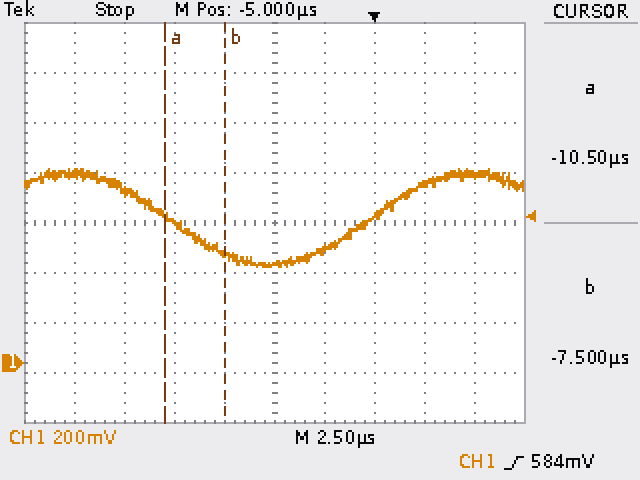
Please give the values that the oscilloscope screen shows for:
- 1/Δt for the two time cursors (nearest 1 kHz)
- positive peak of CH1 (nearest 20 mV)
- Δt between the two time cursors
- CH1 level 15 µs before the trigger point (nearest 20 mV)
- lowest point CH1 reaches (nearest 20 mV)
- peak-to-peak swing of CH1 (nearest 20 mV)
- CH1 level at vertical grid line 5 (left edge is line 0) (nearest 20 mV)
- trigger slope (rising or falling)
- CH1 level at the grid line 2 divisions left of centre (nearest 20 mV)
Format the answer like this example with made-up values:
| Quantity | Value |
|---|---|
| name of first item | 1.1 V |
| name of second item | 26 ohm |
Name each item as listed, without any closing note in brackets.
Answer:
| Quantity | Value |
|---|---|
| 1/Δt for the two time cursors | 333 kHz |
| positive peak of CH1 | 780 mV |
| Δt between the two time cursors | 3.00 µs |
| CH1 level 15 µs before the trigger point | 760 mV |
| lowest point CH1 reaches | 380 mV |
| peak-to-peak swing of CH1 | 400 mV |
| CH1 level at vertical grid line 5 (left edge is line 0) | 400 mV |
| trigger slope | rising |
| CH1 level at the grid line 2 divisions left of centre | 560 mV |
